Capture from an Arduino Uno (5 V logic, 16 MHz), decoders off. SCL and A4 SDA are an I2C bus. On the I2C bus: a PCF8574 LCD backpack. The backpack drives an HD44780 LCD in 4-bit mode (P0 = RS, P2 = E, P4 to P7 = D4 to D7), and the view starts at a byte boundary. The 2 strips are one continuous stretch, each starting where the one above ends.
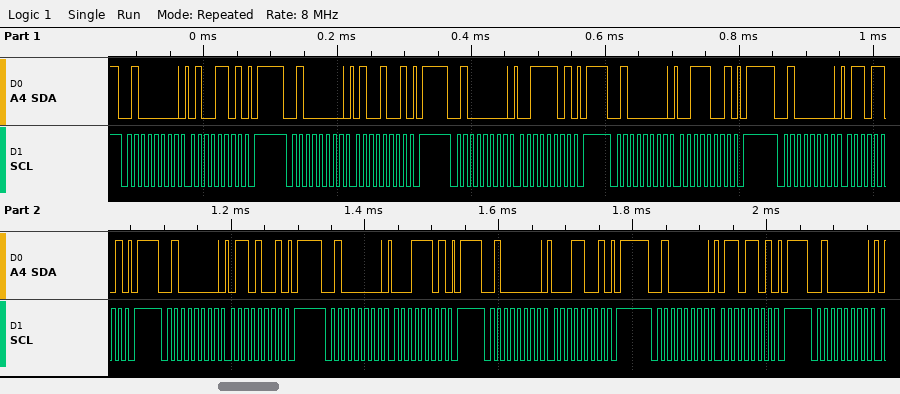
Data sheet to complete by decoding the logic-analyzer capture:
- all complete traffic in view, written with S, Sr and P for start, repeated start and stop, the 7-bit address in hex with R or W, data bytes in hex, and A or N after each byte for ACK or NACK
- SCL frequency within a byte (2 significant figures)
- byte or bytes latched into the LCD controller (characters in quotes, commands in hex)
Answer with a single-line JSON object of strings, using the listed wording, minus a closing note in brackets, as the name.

{"all complete traffic in view, written with S, Sr and P for start, repeated start and stop, the 7-bit address in hex with R or W, data bytes in hex, and A or N after each byte for ACK or NACK": "S 20W A 4D A P S 20W A 49 A P S 20W A 3D A P S 20W A 39 A P S 20W A 6D A P S 20W A 69 A P S 20W A 1D A P S 20W A 19 A P S 20W A 6D A P S 20W A", "SCL frequency within a byte": "100 kHz", "byte or bytes latched into the LCD controller": "'C' 'a'"}
